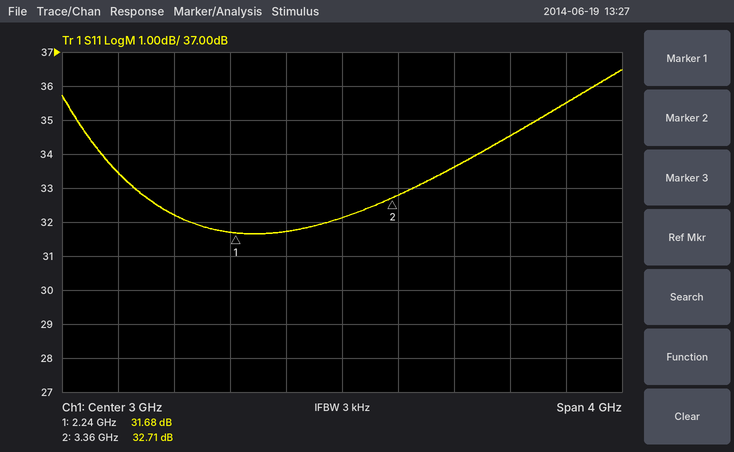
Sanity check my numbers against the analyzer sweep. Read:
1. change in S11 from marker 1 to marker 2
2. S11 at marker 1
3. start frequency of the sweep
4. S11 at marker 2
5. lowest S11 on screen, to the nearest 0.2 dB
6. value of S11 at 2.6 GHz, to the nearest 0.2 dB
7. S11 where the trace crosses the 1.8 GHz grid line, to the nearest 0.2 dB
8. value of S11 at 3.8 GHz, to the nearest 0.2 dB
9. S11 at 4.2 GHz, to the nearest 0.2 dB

1.03 dB
31.68 dB
1 GHz
32.71 dB
31.6 dB
31.8 dB
32.2 dB
33.6 dB
34.6 dB
